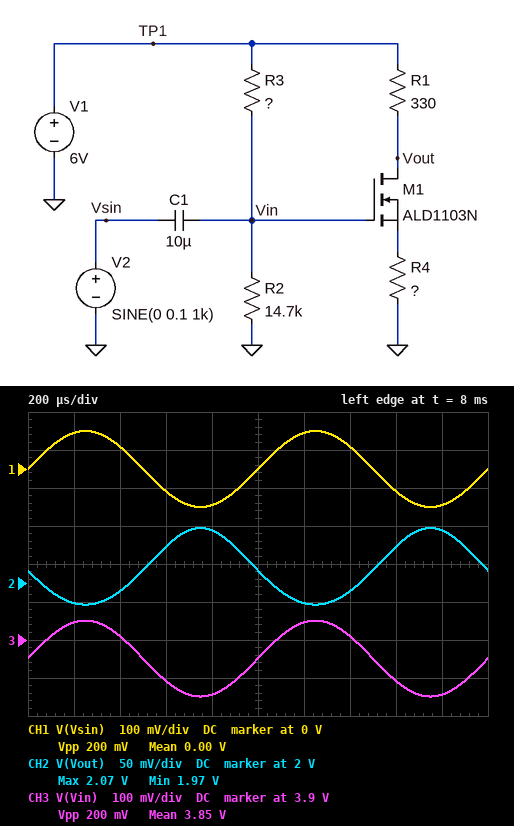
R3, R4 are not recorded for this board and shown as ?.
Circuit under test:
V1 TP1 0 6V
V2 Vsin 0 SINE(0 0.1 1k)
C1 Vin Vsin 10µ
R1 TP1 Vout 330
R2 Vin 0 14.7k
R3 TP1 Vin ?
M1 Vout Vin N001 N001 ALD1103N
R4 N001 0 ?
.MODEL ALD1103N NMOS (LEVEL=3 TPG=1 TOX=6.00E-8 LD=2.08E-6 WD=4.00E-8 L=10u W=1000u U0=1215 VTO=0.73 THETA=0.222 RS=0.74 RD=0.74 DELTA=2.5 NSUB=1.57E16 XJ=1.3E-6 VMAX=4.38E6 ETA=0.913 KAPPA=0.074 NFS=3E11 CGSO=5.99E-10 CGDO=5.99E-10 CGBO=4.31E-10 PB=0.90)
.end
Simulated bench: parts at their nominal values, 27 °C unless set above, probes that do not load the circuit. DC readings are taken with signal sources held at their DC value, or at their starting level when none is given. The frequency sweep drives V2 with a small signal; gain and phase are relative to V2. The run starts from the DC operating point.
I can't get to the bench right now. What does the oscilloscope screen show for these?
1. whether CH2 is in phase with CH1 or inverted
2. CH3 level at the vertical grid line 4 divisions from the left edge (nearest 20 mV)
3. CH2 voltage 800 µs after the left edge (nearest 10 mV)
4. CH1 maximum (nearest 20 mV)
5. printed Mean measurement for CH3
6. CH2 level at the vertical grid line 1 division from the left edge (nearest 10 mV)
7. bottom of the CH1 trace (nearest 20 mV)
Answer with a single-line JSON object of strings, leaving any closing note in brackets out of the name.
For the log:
{"whether CH2 is in phase with CH1 or inverted": "inverted", "CH3 level at the vertical grid line 4 divisions from the left edge": "3.76 V", "CH2 voltage 800 µs after the left edge": "2.07 V", "CH1 maximum": "100 mV", "printed Mean measurement for CH3": "3.85 V", "CH2 level at the vertical grid line 1 division from the left edge": "1.97 V", "bottom of the CH1 trace": "-100 mV"}
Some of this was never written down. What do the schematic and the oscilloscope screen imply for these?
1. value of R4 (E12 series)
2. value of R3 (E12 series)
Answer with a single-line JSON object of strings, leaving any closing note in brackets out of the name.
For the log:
{"value of R4": "82 Ω", "value of R3": "8.2 kΩ"}
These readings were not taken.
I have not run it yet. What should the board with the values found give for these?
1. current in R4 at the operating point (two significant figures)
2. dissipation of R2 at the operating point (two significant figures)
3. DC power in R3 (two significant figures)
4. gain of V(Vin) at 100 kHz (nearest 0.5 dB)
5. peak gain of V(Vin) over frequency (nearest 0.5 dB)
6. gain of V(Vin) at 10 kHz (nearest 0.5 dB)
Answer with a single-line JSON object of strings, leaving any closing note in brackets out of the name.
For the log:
{"current in R4 at the operating point": "12 mA", "dissipation of R2 at the operating point": "1.0 mW", "DC power in R3": "560 µW", "gain of V(Vin) at 100 kHz": "0 dB", "peak gain of V(Vin) over frequency": "0 dB", "gain of V(Vin) at 10 kHz": "0 dB"}
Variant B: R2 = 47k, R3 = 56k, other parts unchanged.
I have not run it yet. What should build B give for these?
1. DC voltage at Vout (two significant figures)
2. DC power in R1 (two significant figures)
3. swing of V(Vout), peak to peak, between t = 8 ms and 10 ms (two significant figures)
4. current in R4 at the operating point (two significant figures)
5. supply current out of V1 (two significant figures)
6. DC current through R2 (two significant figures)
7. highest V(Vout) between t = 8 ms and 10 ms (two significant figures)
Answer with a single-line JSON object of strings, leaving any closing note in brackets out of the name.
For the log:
{"DC voltage at Vout": "3.6 V", "DC power in R1": "17 mW", "swing of V(Vout), peak to peak, between t = 8 ms and 10 ms": "330 mV", "current in R4 at the operating point": "7.2 mA", "supply current out of V1": "7.3 mA", "DC current through R2": "58 µA", "highest V(Vout) between t = 8 ms and 10 ms": "3.8 V"}
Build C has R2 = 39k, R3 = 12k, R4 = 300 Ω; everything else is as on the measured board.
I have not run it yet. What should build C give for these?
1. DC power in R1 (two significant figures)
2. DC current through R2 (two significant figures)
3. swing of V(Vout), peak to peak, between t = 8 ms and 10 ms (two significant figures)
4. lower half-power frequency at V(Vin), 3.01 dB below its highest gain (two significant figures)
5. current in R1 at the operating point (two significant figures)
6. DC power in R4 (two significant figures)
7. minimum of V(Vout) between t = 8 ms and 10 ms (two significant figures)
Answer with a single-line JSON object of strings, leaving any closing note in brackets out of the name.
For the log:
{"DC power in R1": "20 mW", "DC current through R2": "120 µA", "swing of V(Vout), peak to peak, between t = 8 ms and 10 ms": "130 mV", "lower half-power frequency at V(Vin), 3.01 dB below its highest gain": "1.7 Hz", "current in R1 at the operating point": "7.8 mA", "DC power in R4": "18 mW", "minimum of V(Vout) between t = 8 ms and 10 ms": "3.4 V"}
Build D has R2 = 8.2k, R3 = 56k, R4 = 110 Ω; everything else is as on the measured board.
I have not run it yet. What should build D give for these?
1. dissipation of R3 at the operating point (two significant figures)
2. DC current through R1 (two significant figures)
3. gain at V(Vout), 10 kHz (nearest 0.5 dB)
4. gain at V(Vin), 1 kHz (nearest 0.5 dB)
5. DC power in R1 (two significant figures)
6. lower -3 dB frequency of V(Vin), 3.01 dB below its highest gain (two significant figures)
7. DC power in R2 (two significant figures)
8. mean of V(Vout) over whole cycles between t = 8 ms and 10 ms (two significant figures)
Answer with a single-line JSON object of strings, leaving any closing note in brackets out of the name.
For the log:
{"dissipation of R3 at the operating point": "490 µW", "DC current through R1": "55 µA", "gain at V(Vout), 10 kHz": "-11.0 dB", "gain at V(Vin), 1 kHz": "0 dB", "DC power in R1": "1.0 µW", "lower -3 dB frequency of V(Vin), 3.01 dB below its highest gain": "2.2 Hz", "DC power in R2": "72 µW", "mean of V(Vout) over whole cycles between t = 8 ms and 10 ms": "6.0 V"}
